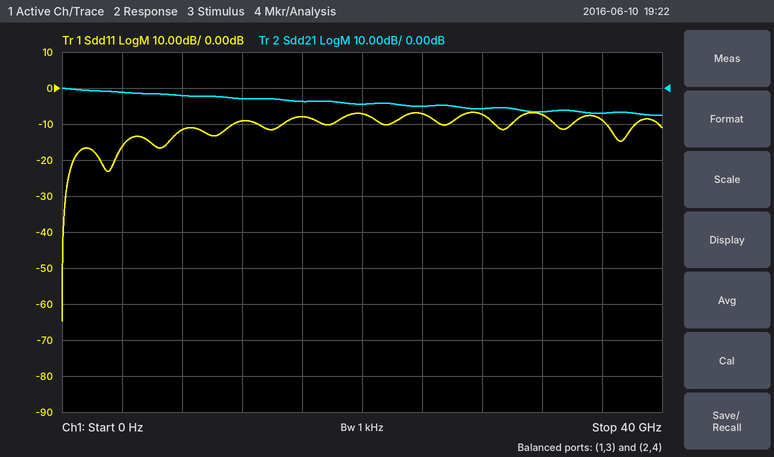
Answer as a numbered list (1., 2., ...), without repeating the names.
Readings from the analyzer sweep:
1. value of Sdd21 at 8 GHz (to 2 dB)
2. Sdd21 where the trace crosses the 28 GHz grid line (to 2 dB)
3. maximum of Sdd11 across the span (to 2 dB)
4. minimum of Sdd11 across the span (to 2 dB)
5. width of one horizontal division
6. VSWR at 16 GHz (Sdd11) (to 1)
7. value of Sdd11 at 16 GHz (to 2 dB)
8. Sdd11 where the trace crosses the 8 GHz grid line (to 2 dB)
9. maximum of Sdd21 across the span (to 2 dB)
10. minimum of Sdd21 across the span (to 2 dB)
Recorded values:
1. -2 dB
2. -6 dB
3. -6 dB
4. -64 dB
5. 4 GHz
6. 2
7. -8 dB
8. -12 dB
9. 0 dB
10. -8 dB
